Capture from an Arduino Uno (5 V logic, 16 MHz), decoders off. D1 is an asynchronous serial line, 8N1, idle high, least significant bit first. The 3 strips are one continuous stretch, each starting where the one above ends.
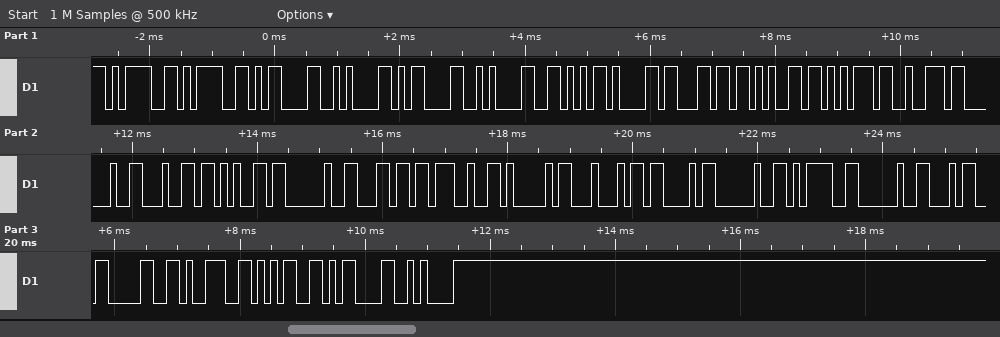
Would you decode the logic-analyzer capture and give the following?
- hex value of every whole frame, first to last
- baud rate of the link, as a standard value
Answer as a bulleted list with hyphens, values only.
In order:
- 3D 3D 0D 0A 0D 0A 56 61 6C 65 75 72 20 64 65 20 6C 27 41 44 43 20 3D 20 34 30 39 35 0D 0A
- 9600 baud
